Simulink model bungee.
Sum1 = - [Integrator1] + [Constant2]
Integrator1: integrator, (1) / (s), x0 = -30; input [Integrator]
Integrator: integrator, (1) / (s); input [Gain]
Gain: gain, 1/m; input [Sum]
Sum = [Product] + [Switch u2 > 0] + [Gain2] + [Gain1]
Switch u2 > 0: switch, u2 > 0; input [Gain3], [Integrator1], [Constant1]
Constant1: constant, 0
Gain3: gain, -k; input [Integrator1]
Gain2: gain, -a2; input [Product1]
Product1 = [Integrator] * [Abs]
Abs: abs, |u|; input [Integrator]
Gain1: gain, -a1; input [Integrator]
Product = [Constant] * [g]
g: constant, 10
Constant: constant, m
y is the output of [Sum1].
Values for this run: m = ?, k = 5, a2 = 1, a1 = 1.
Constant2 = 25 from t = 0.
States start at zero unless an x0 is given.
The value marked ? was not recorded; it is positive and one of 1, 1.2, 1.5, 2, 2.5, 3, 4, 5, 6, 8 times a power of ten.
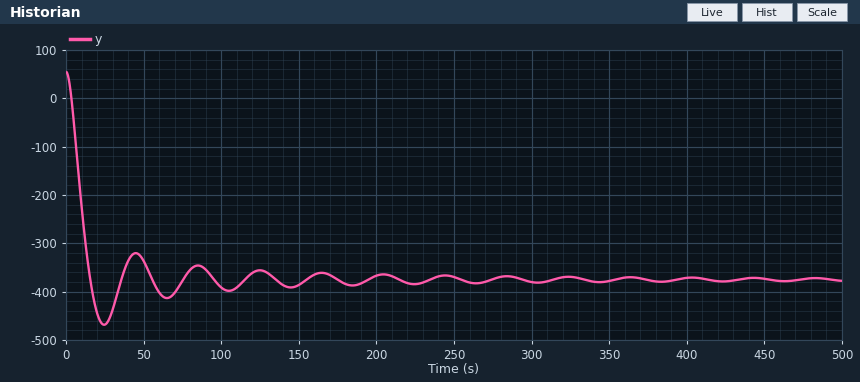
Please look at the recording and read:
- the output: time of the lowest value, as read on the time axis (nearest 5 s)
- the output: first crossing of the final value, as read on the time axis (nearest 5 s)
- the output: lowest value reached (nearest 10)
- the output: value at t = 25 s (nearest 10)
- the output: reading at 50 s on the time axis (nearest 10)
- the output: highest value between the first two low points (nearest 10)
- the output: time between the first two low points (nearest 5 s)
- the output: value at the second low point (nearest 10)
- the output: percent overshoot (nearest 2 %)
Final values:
25 s
15 s
-470
-470
-340
-320
40 s
-410
22 %
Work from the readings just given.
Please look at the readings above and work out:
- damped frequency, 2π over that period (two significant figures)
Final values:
0.16 rad/s
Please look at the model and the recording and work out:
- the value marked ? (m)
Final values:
200
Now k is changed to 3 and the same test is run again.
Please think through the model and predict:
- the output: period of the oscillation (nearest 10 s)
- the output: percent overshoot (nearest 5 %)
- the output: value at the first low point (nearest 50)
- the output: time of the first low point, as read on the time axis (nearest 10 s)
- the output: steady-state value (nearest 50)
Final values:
50 s
15 %
-750
40 s
-650
